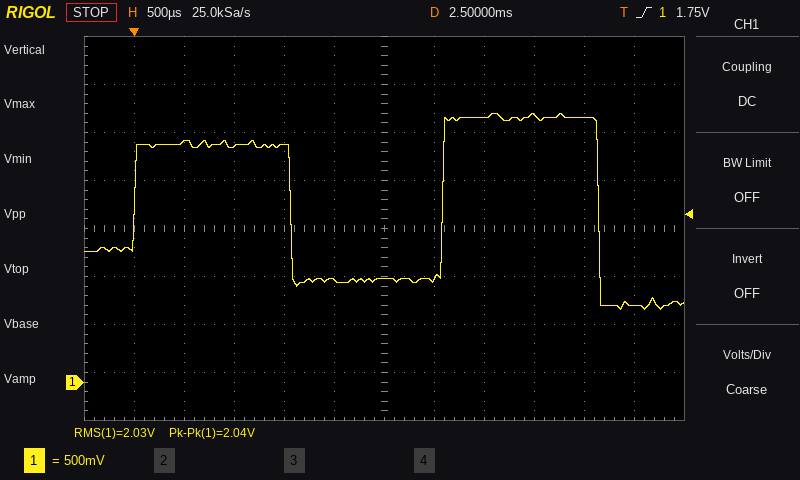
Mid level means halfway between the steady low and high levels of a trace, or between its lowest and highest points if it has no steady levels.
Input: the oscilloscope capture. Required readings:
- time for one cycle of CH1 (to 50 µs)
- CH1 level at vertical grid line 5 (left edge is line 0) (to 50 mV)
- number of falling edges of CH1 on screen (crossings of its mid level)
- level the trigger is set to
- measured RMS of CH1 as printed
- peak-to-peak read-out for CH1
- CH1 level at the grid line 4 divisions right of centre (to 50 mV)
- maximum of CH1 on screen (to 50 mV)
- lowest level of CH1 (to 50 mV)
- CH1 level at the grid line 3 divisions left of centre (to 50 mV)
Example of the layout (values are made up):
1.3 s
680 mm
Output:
3.10 ms
1.05 V
2
1.75 V
2.03 V
2.04 V
2.75 V
2.80 V
750 mV
2.45 V
